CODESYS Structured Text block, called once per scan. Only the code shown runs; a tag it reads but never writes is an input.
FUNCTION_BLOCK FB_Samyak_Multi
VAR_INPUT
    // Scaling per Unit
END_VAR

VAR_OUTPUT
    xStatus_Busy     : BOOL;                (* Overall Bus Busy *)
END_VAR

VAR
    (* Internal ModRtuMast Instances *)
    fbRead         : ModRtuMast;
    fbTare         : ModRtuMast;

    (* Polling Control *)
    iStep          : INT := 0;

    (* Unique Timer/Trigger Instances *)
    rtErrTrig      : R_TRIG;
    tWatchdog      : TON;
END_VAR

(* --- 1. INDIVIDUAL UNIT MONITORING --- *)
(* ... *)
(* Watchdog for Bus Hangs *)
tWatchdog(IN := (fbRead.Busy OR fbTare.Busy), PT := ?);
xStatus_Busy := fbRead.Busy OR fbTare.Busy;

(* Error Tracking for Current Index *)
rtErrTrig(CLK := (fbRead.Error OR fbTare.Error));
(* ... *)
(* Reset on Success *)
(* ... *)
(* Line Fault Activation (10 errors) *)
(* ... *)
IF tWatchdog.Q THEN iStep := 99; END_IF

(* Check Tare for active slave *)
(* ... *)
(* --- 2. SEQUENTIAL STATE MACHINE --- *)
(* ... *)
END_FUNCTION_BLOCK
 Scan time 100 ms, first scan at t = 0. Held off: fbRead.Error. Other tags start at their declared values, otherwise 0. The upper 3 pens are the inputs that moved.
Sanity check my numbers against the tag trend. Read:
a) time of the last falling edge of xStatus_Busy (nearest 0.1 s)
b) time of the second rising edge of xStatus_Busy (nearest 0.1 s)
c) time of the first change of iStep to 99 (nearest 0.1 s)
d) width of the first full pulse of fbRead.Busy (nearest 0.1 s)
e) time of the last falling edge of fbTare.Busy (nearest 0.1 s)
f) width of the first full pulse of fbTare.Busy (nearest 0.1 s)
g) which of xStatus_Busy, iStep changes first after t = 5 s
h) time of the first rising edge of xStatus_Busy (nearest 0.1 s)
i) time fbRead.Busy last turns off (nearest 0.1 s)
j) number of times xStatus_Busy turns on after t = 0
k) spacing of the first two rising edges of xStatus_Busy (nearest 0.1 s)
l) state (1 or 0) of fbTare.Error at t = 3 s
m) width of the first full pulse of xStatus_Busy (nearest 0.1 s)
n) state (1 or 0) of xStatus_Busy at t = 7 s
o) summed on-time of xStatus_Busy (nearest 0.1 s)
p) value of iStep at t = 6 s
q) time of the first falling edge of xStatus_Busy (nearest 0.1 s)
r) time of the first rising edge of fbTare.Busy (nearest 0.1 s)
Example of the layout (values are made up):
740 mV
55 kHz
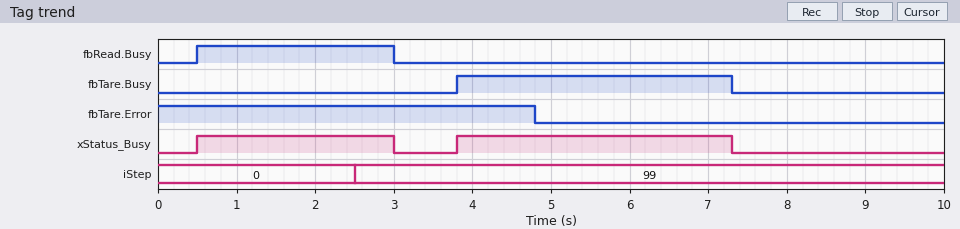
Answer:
7.3 s
3.8 s
2.5 s
2.5 s
7.3 s
3.5 s
xStatus_Busy
0.5 s
3.0 s
2
3.3 s
1
2.5 s
1
6.0 s
99
3.0 s
3.8 s
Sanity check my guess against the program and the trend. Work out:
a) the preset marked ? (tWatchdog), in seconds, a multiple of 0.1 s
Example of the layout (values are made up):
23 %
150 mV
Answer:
2.0 s
